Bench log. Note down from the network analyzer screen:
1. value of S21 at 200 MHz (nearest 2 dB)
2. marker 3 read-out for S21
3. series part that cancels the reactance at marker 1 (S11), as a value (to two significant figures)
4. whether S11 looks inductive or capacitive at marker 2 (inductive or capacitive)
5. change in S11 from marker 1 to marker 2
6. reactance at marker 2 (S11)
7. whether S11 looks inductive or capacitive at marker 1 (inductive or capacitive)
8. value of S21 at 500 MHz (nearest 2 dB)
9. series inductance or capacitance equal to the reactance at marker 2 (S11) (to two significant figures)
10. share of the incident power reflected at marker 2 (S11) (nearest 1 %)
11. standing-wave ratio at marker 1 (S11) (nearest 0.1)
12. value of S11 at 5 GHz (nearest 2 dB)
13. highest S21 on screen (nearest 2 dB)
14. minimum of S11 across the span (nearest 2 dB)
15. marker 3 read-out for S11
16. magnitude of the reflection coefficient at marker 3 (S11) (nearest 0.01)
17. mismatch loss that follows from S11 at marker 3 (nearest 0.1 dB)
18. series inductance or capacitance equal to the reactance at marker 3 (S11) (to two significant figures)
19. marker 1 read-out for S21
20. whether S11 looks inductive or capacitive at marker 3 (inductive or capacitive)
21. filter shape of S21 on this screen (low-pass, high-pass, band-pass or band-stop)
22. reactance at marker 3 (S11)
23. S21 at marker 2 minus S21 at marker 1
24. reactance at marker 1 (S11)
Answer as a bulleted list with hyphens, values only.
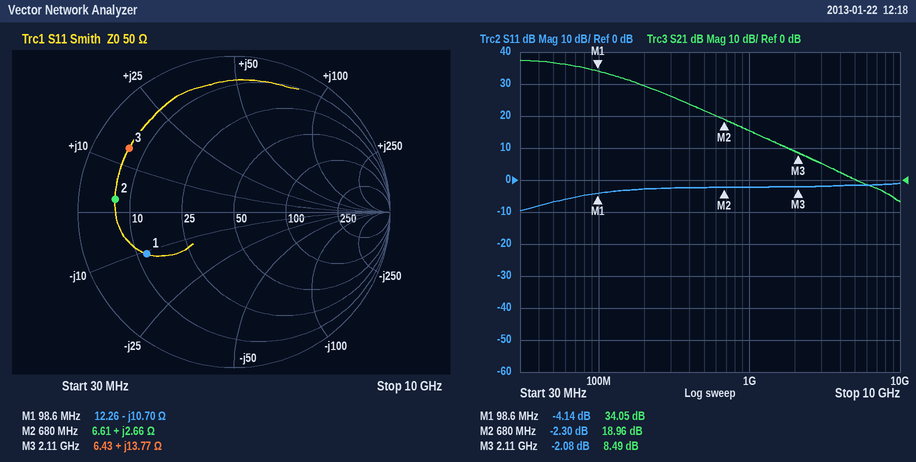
- 30 dB
- 8.49 dB
- 17 nH
- inductive
- 1.84 dB
- +2.66 Ω
- capacitive
- 22 dB
- 620 pH
- 59 %
- 4.3
- -2 dB
- 38 dB
- -10 dB
- -2.08 dB
- 0.79
- 4.2 dB
- 1.0 nH
- 34.05 dB
- inductive
- low-pass
- +13.77 Ω
- -15.09 dB
- -10.70 Ω
